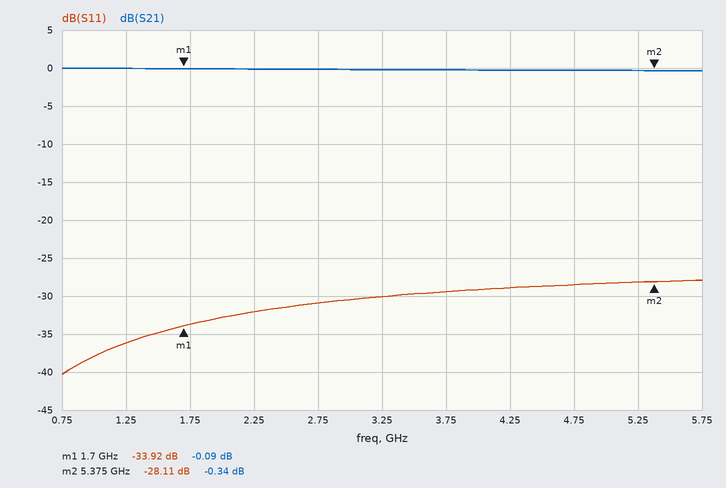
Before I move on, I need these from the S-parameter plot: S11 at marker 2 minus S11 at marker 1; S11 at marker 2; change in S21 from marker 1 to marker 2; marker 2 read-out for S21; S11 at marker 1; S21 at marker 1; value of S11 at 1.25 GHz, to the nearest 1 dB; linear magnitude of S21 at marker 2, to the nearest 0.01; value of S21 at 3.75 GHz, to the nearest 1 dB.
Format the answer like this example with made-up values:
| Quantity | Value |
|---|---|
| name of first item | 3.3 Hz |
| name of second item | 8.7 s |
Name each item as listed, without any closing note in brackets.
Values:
| Quantity | Value |
|---|---|
| S11 at marker 2 minus S11 at marker 1 | 5.81 dB |
| S11 at marker 2 | -28.11 dB |
| change in S21 from marker 1 to marker 2 | -0.25 dB |
| marker 2 read-out for S21 | -0.34 dB |
| S11 at marker 1 | -33.92 dB |
| S21 at marker 1 | -0.09 dB |
| value of S11 at 1.25 GHz, to the nearest 1 dB | -36 dB |
| linear magnitude of S21 at marker 2, to the nearest 0.01 | 0.96 |
| value of S21 at 3.75 GHz, to the nearest 1 dB | 0 dB |
